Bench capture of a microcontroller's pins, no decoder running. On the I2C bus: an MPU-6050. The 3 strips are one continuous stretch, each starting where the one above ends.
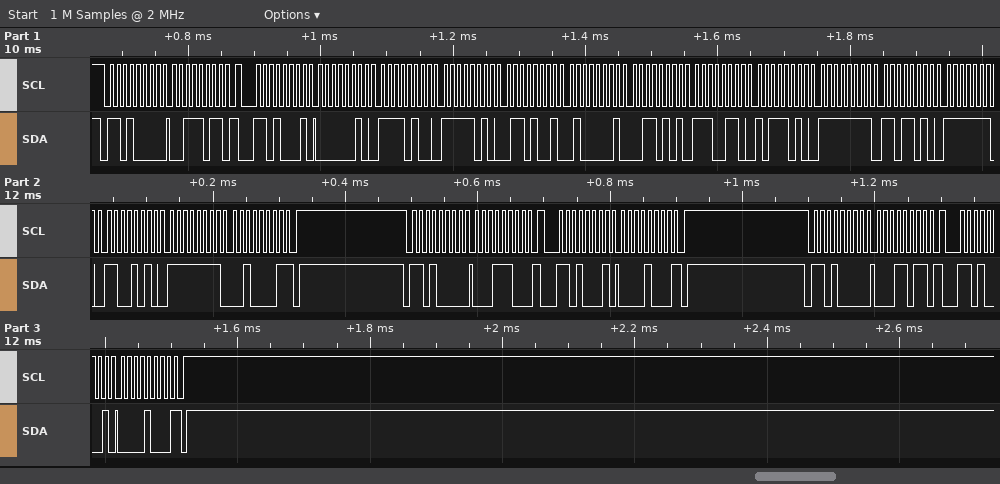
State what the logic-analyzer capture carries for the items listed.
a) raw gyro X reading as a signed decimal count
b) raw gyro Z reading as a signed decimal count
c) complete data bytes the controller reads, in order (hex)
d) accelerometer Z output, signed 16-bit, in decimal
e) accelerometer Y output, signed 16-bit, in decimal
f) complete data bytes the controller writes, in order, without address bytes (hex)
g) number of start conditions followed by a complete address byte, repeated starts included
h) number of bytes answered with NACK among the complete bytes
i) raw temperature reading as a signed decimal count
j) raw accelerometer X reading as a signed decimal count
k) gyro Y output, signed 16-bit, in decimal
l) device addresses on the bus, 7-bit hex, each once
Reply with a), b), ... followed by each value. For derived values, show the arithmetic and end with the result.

a) 0xFFDA = -38
b) 0xFF21 = -223
c) 02 F4 FA 69 41 35 E6 BA FF DA FE CA FF 21 08 08
d) 0x4135 = 16693
e) 0xFA69 = -1431
f) 3B 1C 1B
g) 6
h) 3
i) 0xE6BA = -6470
j) 0x02F4 = 756
k) 0xFECA = -310
l) 0x68
